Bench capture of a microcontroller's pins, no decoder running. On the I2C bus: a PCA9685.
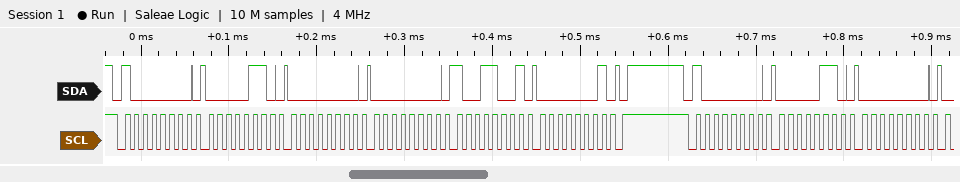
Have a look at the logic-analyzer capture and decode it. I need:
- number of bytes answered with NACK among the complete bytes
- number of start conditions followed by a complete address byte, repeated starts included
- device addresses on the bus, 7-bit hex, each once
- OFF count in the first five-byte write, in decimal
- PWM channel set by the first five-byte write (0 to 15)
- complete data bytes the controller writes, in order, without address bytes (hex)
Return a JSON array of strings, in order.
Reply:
["0", "2", "0x40", "409", "0", "06 00 00 99 01 06 00"]
